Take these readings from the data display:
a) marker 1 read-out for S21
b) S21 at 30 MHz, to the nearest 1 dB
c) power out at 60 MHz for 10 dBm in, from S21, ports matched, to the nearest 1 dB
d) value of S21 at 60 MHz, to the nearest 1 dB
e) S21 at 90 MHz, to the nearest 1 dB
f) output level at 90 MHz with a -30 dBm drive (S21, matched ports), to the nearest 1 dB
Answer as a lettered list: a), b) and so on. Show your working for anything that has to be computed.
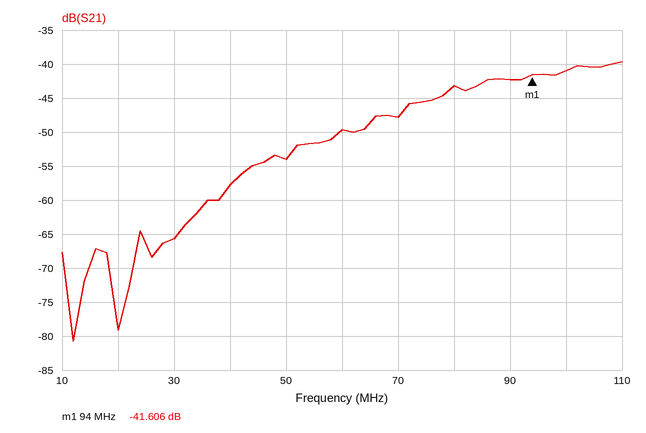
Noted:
a) -41.606 dB
b) -66 dB
c) 10 dBm + (-50 dB) = -40 dBm
d) -50 dB
e) -42 dB
f) -30 dBm + (-42 dB) = -72 dBm
